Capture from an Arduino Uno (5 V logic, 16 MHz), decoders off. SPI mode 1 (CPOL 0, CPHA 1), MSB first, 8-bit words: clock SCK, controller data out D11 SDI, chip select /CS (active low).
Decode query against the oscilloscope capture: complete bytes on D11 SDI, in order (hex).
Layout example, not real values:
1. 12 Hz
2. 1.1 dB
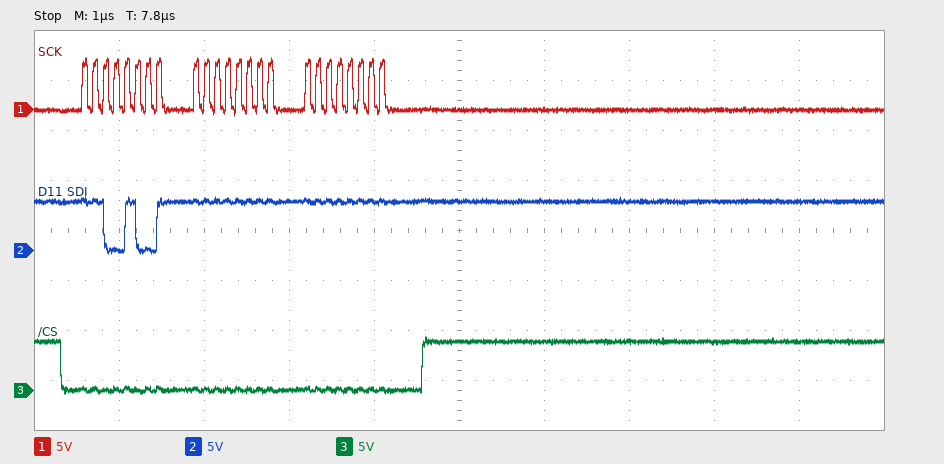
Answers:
1. 0xC9 0xFF 0xFF
